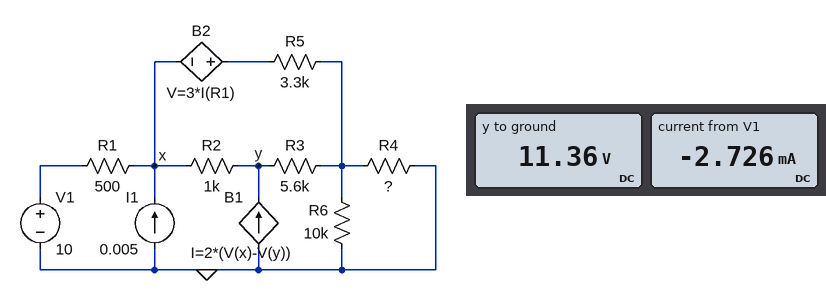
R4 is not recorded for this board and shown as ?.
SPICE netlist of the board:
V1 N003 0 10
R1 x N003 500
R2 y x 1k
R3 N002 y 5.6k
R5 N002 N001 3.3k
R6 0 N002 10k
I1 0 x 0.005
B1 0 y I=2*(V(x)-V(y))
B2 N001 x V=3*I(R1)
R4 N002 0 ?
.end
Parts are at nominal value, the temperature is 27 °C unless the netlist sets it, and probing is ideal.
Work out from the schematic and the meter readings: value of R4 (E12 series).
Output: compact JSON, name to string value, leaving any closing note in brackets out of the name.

{"value of R4": "1.2 kΩ"}
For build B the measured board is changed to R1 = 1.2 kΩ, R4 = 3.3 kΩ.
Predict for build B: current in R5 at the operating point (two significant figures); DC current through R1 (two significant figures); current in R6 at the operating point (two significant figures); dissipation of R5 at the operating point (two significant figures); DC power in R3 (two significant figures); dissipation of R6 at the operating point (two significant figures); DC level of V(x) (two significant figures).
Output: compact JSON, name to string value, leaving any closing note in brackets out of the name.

{"current in R5 at the operating point": "1.9 mA", "DC current through R1": "3.1 mA", "current in R6 at the operating point": "750 µA", "dissipation of R5 at the operating point": "12 mW", "DC power in R3": "7.0 mW", "dissipation of R6 at the operating point": "5.6 mW", "DC level of V(x)": "14 V"}
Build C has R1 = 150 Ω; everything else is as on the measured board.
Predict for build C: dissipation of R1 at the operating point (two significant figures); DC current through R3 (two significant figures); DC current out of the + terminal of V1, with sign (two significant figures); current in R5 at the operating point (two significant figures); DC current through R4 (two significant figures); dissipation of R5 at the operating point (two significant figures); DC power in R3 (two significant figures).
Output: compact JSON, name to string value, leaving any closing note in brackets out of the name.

{"dissipation of R1 at the operating point": "1.3 mW", "DC current through R3": "1.2 mA", "DC current out of the + terminal of V1, with sign": "-2.9 mA", "current in R5 at the operating point": "2.1 mA", "DC current through R4": "3.0 mA", "dissipation of R5 at the operating point": "14 mW", "DC power in R3": "8.5 mW"}
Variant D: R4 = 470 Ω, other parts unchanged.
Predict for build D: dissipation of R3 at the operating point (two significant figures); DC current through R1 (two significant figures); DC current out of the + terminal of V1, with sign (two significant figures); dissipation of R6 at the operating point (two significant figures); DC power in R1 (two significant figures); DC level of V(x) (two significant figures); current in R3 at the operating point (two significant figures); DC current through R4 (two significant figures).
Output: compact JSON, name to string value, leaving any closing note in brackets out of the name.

{"dissipation of R3 at the operating point": "15 mW", "DC current through R1": "2.2 mA", "DC current out of the + terminal of V1, with sign": "-2.2 mA", "dissipation of R6 at the operating point": "390 µW", "DC power in R1": "2.5 mW", "DC level of V(x)": "11 V", "current in R3 at the operating point": "1.6 mA", "DC current through R4": "4.2 mA"}
